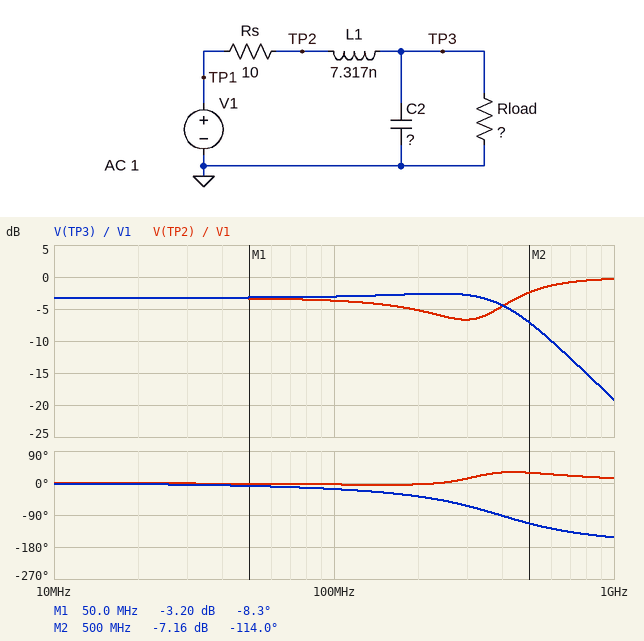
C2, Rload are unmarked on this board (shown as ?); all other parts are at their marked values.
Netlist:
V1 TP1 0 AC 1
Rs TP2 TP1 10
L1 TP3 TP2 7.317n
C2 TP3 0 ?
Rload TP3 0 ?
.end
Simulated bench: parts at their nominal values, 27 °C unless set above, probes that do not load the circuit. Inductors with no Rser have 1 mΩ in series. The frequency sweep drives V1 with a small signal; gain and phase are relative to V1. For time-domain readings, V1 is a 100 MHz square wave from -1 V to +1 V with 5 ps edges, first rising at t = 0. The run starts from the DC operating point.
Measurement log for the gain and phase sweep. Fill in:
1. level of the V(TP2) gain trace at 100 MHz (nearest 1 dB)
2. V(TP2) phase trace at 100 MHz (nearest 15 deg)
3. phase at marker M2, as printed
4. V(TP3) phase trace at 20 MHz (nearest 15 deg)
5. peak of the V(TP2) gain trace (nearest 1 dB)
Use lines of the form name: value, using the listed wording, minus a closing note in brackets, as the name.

level of the V(TP2) gain trace at 100 MHz: -4 dB
V(TP2) phase trace at 100 MHz: 0 deg
phase at marker M2, as printed: -114.0 deg
V(TP3) phase trace at 20 MHz: 0 deg
peak of the V(TP2) gain trace: 0 dB
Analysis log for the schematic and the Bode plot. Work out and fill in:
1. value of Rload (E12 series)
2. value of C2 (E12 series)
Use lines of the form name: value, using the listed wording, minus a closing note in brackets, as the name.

value of Rload: 22 Ω
value of C2: 33 pF
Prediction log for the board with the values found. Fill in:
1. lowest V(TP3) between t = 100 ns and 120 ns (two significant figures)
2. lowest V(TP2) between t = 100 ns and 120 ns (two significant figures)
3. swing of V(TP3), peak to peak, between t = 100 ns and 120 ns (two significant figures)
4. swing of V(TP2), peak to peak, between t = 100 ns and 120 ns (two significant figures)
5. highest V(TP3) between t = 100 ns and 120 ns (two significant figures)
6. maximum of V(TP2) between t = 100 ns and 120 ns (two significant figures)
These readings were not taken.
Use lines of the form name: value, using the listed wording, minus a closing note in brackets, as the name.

lowest V(TP3) between t = 100 ns and 120 ns: -850 mV
lowest V(TP2) between t = 100 ns and 120 ns: -1.3 V
swing of V(TP3), peak to peak, between t = 100 ns and 120 ns: 1.7 V
swing of V(TP2), peak to peak, between t = 100 ns and 120 ns: 2.6 V
highest V(TP3) between t = 100 ns and 120 ns: 850 mV
maximum of V(TP2) between t = 100 ns and 120 ns: 1.3 V
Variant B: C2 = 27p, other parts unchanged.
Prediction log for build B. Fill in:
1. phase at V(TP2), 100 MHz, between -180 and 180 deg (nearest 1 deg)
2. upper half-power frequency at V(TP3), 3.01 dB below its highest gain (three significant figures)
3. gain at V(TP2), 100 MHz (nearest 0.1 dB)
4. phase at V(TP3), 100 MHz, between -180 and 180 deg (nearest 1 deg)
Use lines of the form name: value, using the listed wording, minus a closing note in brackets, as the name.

phase at V(TP2), 100 MHz, between -180 and 180 deg: -3 deg
upper half-power frequency at V(TP3), 3.01 dB below its highest gain: 492 MHz
gain at V(TP2), 100 MHz: -3.6 dB
phase at V(TP3), 100 MHz, between -180 and 180 deg: -15 deg
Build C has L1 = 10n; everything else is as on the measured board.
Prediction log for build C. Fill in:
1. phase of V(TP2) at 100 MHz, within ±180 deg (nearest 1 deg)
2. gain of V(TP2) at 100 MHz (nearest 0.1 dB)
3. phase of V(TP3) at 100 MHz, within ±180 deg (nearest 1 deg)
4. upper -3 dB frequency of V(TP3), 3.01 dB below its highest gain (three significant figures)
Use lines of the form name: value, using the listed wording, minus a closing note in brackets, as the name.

phase of V(TP2) at 100 MHz, within ±180 deg: -2 deg
gain of V(TP2) at 100 MHz: -3.8 dB
phase of V(TP3) at 100 MHz, within ±180 deg: -20 deg
upper -3 dB frequency of V(TP3), 3.01 dB below its highest gain: 380 MHz
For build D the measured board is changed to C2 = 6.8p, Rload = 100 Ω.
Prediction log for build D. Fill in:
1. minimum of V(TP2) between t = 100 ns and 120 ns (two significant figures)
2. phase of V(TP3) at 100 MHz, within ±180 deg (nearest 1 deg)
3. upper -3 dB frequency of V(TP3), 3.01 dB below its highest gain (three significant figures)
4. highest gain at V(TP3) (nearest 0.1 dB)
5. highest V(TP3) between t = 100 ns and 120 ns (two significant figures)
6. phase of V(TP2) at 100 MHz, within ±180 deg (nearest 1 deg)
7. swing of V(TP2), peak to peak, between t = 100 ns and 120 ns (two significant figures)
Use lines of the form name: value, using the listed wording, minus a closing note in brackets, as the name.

minimum of V(TP2) between t = 100 ns and 120 ns: -1.1 V
phase of V(TP3) at 100 MHz, within ±180 deg: -5 deg
upper -3 dB frequency of V(TP3), 3.01 dB below its highest gain: 883 MHz
highest gain at V(TP3): 4.0 dB
highest V(TP3) between t = 100 ns and 120 ns: 1.6 V
phase of V(TP2) at 100 MHz, within ±180 deg: -2 deg
swing of V(TP2), peak to peak, between t = 100 ns and 120 ns: 2.2 V
